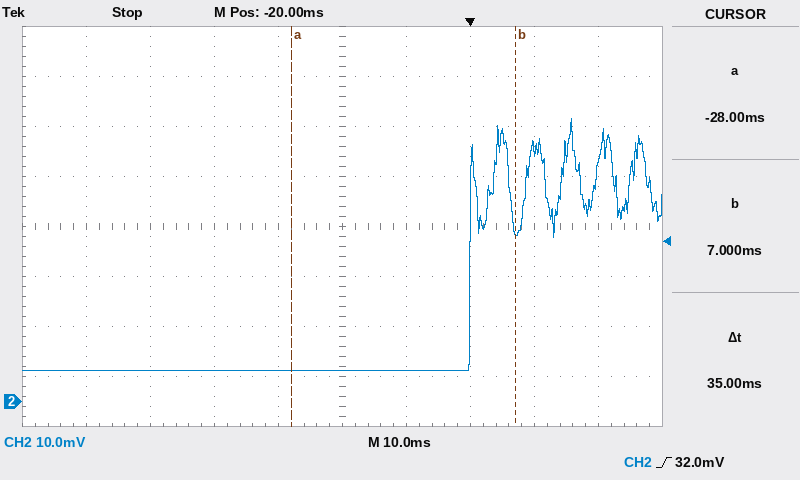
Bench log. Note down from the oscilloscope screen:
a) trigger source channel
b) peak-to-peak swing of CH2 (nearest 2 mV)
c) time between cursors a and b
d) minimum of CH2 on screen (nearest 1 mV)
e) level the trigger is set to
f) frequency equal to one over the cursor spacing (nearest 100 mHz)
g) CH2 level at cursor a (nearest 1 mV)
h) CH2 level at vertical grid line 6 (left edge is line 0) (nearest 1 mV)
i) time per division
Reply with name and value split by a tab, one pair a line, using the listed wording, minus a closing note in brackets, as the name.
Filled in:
trigger source channel	CH2
peak-to-peak swing of CH2	50 mV
time between cursors a and b	35 ms
minimum of CH2 on screen	6 mV
level the trigger is set to	32.0 mV
frequency equal to one over the cursor spacing	28.6 Hz
CH2 level at cursor a	6 mV
CH2 level at vertical grid line 6 (left edge is line 0)	6 mV
time per division	10 ms
